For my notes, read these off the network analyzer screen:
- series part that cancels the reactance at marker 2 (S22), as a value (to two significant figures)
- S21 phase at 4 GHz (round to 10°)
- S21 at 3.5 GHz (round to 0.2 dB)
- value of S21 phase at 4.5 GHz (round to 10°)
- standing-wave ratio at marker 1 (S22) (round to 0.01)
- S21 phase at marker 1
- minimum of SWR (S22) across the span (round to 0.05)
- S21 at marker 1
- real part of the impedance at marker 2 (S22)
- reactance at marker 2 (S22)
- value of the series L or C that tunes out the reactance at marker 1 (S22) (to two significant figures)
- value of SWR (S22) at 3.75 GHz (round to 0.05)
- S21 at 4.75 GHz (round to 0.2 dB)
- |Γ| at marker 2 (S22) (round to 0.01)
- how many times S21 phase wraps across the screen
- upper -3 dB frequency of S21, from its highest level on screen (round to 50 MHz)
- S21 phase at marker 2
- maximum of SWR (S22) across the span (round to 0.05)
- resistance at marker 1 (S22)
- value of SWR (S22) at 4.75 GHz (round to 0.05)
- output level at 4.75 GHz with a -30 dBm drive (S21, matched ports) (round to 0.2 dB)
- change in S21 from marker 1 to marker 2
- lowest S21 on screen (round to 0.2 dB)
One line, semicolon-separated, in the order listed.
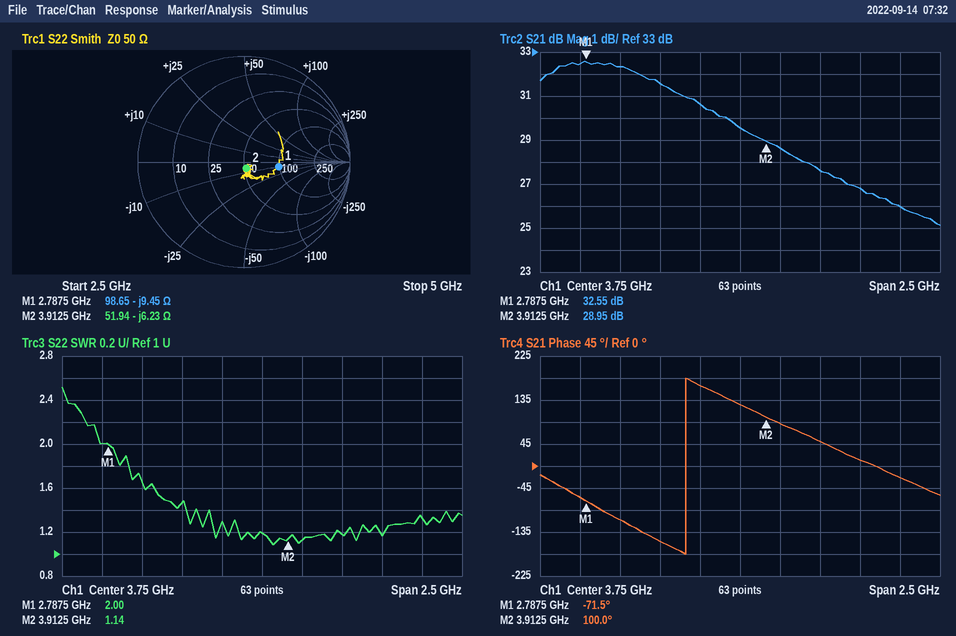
250 pH; 90°; 30.6 dB; 10°; 2.00; -71.5°; 1.10; 32.55 dB; 51.94 Ω; -6.23 Ω; 540 pH; 1.20; 26.0 dB; 0.06; 1; 3.75 GHz; 100.0°; 2.50; 98.65 Ω; 1.35; -4.0 dBm; -3.60 dB; 25.2 dB
